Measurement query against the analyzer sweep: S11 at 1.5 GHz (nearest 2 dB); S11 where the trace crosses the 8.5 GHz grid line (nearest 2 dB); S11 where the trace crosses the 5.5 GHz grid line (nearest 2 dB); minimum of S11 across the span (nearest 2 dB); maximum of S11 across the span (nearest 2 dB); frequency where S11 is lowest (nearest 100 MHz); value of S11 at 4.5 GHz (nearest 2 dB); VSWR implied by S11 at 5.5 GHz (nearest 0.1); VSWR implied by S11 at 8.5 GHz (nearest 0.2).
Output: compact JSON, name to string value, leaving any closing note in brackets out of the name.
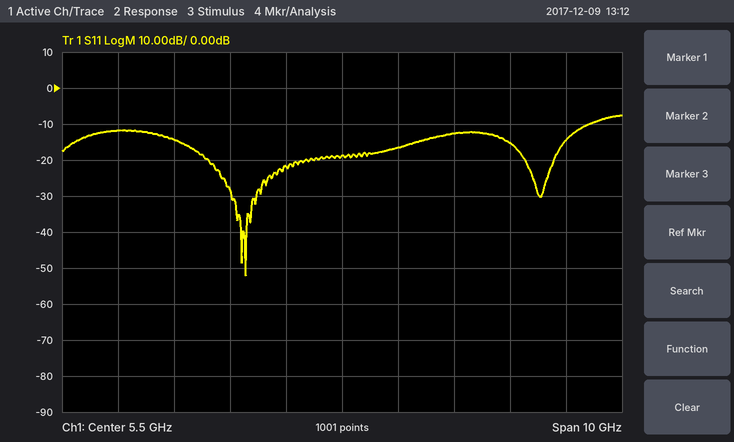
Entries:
{"S11 at 1.5 GHz": "-12 dB", "S11 where the trace crosses the 8.5 GHz grid line": "-16 dB", "S11 where the trace crosses the 5.5 GHz grid line": "-18 dB", "minimum of S11 across the span": "-52 dB", "maximum of S11 across the span": "-8 dB", "frequency where S11 is lowest": "3.8 GHz", "value of S11 at 4.5 GHz": "-22 dB", "VSWR implied by S11 at 5.5 GHz": "1.3", "VSWR implied by S11 at 8.5 GHz": "1.4"}
